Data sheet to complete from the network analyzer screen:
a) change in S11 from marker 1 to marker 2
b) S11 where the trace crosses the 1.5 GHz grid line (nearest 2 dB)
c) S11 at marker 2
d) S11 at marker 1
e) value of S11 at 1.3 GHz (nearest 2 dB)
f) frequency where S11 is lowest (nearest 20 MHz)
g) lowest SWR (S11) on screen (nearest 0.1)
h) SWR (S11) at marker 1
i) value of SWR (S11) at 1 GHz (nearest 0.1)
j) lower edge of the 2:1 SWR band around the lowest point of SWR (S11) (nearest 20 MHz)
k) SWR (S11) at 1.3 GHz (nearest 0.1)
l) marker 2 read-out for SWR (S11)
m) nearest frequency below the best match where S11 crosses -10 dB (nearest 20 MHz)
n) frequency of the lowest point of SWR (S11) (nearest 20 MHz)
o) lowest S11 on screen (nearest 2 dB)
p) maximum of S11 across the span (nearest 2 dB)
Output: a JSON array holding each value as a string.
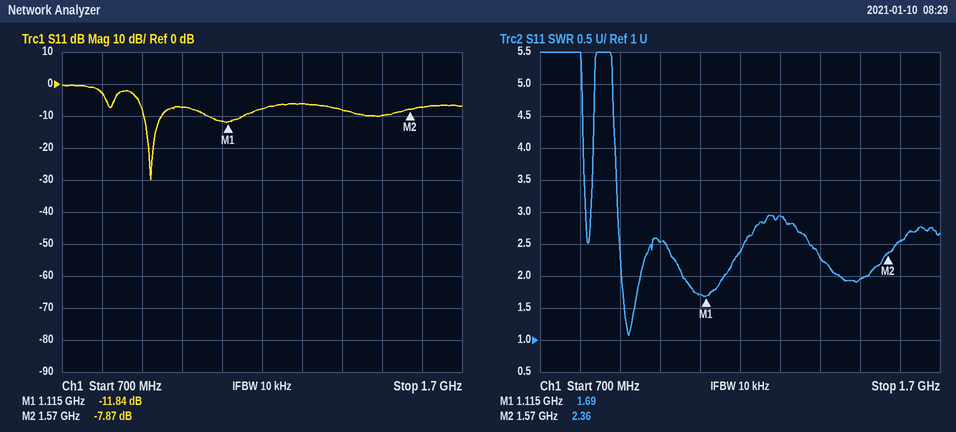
["3.97 dB", "-10 dB", "-7.87 dB", "-11.84 dB", "-6 dB", "920 MHz", "1.1", "1.69", "2.5", "900 MHz", "2.9", "2.36", "900 MHz", "920 MHz", "-30 dB", "0 dB"]
